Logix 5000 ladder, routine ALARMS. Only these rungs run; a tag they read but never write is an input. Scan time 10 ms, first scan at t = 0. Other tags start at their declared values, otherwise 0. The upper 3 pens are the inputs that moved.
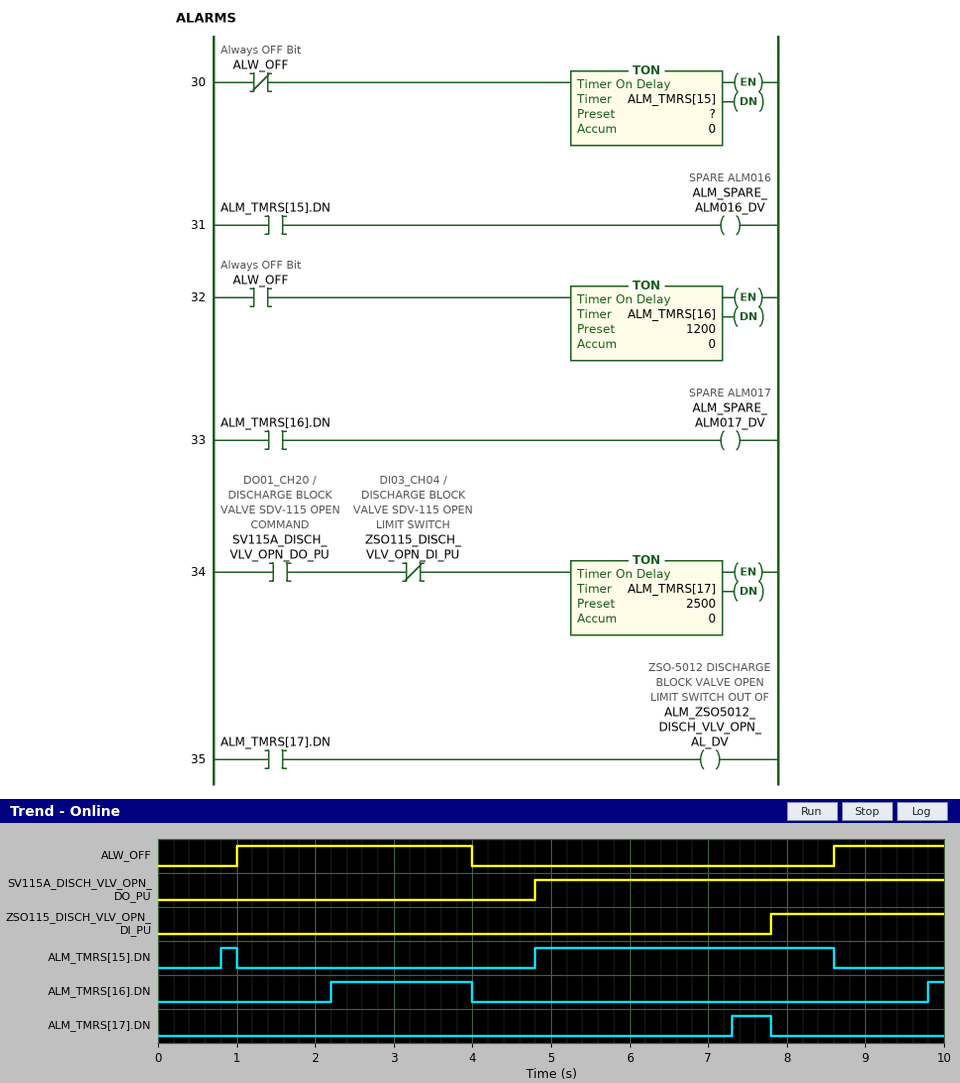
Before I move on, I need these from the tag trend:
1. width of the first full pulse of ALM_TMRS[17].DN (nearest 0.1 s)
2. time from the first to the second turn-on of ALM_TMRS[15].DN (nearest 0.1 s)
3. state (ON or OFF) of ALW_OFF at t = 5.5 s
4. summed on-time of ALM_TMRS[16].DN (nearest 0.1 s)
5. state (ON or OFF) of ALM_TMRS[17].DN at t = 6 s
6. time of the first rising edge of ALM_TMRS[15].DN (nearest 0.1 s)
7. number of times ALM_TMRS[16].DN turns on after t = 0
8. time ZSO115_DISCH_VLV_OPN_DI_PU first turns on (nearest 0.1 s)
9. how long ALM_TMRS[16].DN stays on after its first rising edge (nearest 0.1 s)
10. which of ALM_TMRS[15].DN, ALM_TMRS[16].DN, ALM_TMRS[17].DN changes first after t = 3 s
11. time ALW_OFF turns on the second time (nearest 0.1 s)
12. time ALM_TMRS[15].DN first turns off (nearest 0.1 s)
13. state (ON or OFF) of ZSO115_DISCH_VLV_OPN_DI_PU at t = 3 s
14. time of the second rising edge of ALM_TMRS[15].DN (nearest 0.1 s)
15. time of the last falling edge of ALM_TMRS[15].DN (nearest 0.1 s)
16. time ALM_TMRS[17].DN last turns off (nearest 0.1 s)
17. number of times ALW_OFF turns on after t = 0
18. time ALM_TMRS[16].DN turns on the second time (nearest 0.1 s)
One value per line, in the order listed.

0.5 s
4.0 s
OFF
2.0 s
OFF
0.8 s
2
7.8 s
1.8 s
ALM_TMRS[16].DN
8.6 s
1.0 s
OFF
4.8 s
8.6 s
7.8 s
2
9.8 s
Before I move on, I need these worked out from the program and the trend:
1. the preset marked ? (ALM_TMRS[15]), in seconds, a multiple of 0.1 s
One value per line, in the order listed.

0.8 s
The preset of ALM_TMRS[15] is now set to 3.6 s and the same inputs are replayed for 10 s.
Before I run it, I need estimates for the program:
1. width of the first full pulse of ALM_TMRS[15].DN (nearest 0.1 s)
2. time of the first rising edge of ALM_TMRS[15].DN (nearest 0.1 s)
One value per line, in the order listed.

1.0 s
7.6 s
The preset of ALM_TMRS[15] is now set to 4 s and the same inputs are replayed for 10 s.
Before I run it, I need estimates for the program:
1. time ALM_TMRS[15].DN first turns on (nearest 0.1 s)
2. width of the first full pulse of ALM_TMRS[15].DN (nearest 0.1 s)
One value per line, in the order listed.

8.0 s
0.6 s
